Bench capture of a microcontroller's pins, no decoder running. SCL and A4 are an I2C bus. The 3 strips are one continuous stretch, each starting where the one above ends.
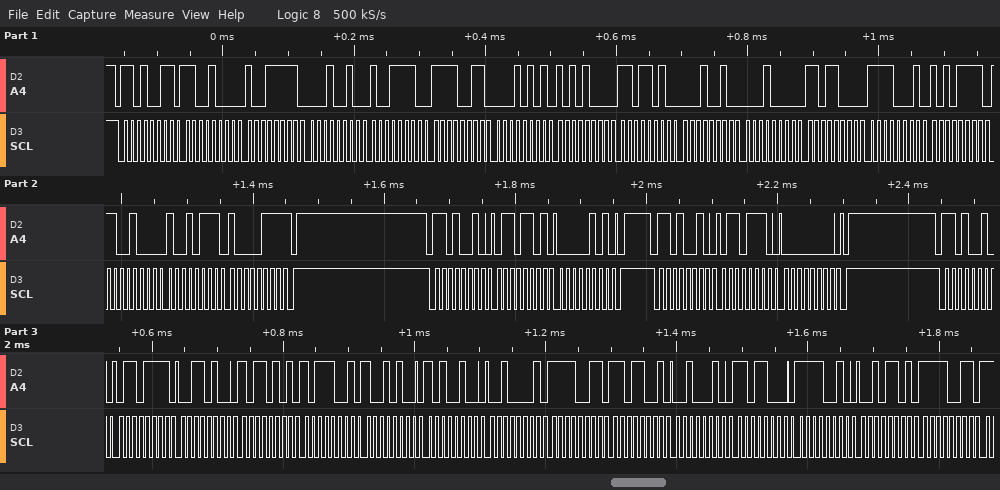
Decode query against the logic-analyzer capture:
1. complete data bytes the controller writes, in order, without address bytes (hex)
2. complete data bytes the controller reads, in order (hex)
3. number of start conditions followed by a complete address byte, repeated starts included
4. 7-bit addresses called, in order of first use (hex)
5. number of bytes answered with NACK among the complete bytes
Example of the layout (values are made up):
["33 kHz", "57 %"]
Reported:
["6D 05 6E 00 6F 34 B5 B9 94 A4 21 F3 D9 22 D8 F2 2D F3", "C8 9F 12 9E F3 15 A8 DA 12 10 D8 F1 AF C8 97 87", "4", "0x69", "1"]
